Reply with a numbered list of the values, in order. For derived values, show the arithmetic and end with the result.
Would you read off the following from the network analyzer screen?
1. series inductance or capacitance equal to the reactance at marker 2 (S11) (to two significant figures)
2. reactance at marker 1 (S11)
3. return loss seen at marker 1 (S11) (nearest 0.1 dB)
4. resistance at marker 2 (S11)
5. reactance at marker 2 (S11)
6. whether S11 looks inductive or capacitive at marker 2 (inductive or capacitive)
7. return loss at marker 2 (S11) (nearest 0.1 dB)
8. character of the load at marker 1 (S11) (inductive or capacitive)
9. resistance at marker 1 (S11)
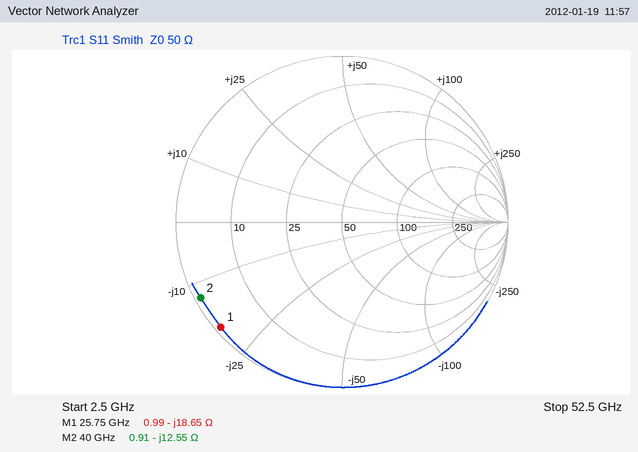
1. C = 1/(2π × 40 GHz × 12.55 Ω) ≈ 317 fF, so 320 fF to two significant figures
2. -18.65 Ω
3. 0.3 dB
4. 0.91 Ω
5. -12.55 Ω
6. capacitive
7. 0.3 dB
8. capacitive
9. 0.99 Ω
